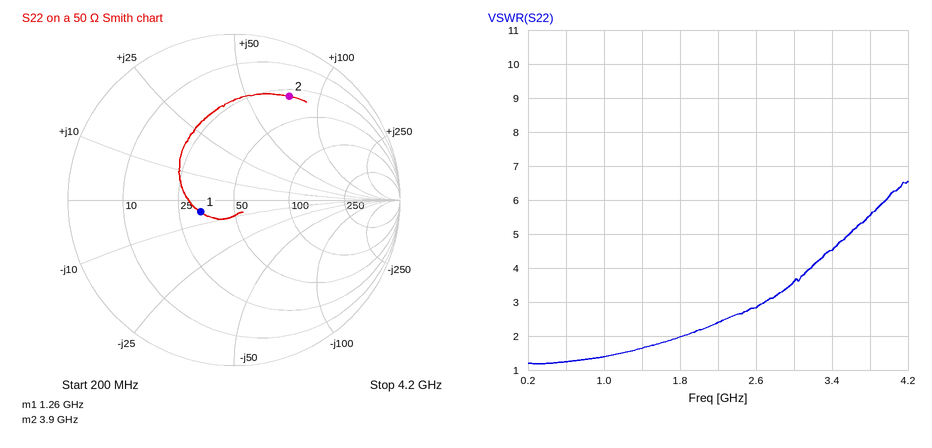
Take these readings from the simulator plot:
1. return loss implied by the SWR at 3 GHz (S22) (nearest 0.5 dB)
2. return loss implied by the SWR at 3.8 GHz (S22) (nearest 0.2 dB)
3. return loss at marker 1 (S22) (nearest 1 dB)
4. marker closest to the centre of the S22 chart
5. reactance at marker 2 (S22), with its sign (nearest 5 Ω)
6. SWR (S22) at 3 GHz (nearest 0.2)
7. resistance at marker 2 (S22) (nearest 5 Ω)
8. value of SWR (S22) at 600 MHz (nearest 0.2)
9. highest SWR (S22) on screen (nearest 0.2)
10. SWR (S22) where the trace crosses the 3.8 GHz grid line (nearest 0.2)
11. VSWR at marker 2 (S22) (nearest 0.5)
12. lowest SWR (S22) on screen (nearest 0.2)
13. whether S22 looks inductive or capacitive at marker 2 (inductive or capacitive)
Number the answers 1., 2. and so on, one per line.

1. 5.0 dB
2. 3.2 dB
3. 13 dB
4. marker 1
5. +75 Ω
6. 3.6
7. 30 Ω
8. 1.2
9. 6.6
10. 5.6
11. 6.0
12. 1.2
13. inductive
